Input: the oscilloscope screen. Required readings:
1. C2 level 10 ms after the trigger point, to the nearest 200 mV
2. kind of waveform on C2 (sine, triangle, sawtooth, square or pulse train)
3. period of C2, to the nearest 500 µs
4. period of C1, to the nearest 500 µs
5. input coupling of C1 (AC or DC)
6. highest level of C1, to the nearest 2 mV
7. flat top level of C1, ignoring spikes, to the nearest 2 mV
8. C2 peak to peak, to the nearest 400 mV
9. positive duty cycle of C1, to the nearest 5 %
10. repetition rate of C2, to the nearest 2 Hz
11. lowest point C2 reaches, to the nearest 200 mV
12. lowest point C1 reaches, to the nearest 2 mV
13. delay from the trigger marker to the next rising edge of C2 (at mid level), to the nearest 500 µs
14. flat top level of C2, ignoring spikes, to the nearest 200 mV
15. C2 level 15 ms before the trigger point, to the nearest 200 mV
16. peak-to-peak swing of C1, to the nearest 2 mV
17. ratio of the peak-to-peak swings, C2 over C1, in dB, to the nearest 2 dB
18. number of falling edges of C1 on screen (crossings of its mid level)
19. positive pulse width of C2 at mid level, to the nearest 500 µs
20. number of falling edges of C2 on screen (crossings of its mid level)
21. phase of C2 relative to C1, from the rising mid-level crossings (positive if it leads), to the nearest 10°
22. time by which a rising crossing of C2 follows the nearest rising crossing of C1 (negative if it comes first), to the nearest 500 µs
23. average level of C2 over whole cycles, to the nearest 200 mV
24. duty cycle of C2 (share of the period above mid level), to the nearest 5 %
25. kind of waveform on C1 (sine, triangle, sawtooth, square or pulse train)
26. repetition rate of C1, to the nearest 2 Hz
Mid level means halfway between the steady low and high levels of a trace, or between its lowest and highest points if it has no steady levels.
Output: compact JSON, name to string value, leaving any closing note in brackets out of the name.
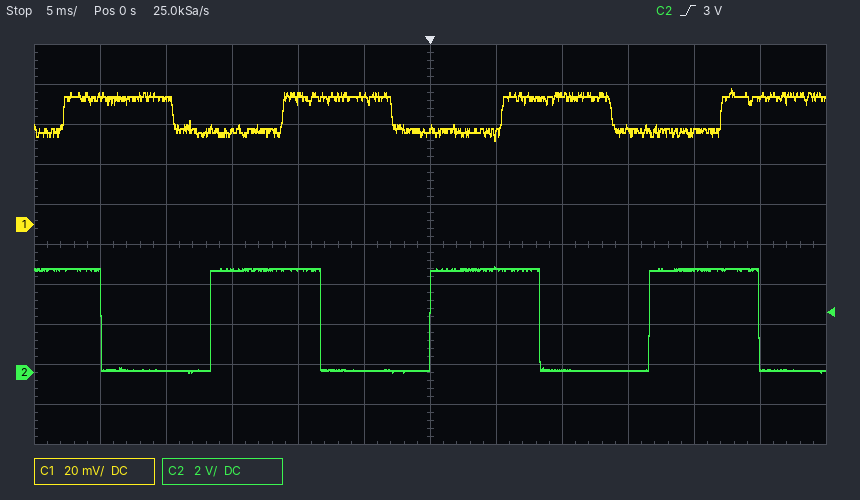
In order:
{"C2 level 10 ms after the trigger point, to the nearest 200 mV": "200 mV", "kind of waveform on C2": "square", "period of C2, to the nearest 500 µs": "16.5 ms", "period of C1, to the nearest 500 µs": "16.5 ms", "input coupling of C1": "DC", "highest level of C1, to the nearest 2 mV": "68 mV", "flat top level of C1, ignoring spikes, to the nearest 2 mV": "64 mV", "C2 peak to peak, to the nearest 400 mV": "5.2 V", "positive duty cycle of C1, to the nearest 5 %": "50 %", "repetition rate of C2, to the nearest 2 Hz": "60 Hz", "lowest point C2 reaches, to the nearest 200 mV": "0.0 V", "lowest point C1 reaches, to the nearest 2 mV": "42 mV", "delay from the trigger marker to the next rising edge of C2 (at mid level), to the nearest 500 µs": "16.5 ms", "flat top level of C2, ignoring spikes, to the nearest 200 mV": "5.2 V", "C2 level 15 ms before the trigger point, to the nearest 200 mV": "5.2 V", "peak-to-peak swing of C1, to the nearest 2 mV": "26 mV", "ratio of the peak-to-peak swings, C2 over C1, in dB, to the nearest 2 dB": "46 dB", "number of falling edges of C1 on screen": "3", "positive pulse width of C2 at mid level, to the nearest 500 µs": "8.5 ms", "number of falling edges of C2 on screen": "4", "phase of C2 relative to C1, from the rising mid-level crossings (positive if it leads), to the nearest 10°": "+120°", "time by which a rising crossing of C2 follows the nearest rising crossing of C1 (negative if it comes first), to the nearest 500 µs": "-5.5 ms", "average level of C2 over whole cycles, to the nearest 200 mV": "2.6 V", "duty cycle of C2 (share of the period above mid level), to the nearest 5 %": "50 %", "kind of waveform on C1": "square", "repetition rate of C1, to the nearest 2 Hz": "60 Hz"}
